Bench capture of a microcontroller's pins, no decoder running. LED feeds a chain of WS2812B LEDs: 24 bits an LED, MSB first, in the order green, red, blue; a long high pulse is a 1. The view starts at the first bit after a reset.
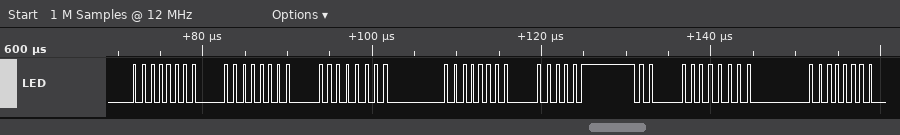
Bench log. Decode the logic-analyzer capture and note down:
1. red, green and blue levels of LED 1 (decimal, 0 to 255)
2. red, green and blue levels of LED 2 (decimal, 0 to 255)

0, 0, 0
4, 0, 0
